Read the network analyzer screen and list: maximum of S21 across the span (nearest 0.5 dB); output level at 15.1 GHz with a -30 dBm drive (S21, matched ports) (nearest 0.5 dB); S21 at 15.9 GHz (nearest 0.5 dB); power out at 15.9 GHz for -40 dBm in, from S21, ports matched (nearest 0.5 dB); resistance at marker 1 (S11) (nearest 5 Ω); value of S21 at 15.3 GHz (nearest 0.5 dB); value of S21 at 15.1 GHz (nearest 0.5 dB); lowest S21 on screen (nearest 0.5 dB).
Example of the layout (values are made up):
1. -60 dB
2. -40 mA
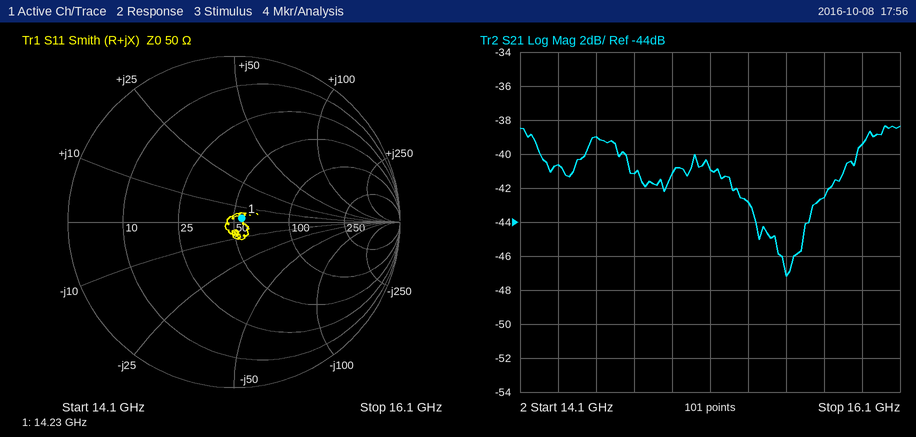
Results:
1. -38.5 dB
2. -71.0 dBm
3. -39.5 dB
4. -79.5 dBm
5. 55 Ω
6. -43.0 dB
7. -41.0 dB
8. -47.0 dB
